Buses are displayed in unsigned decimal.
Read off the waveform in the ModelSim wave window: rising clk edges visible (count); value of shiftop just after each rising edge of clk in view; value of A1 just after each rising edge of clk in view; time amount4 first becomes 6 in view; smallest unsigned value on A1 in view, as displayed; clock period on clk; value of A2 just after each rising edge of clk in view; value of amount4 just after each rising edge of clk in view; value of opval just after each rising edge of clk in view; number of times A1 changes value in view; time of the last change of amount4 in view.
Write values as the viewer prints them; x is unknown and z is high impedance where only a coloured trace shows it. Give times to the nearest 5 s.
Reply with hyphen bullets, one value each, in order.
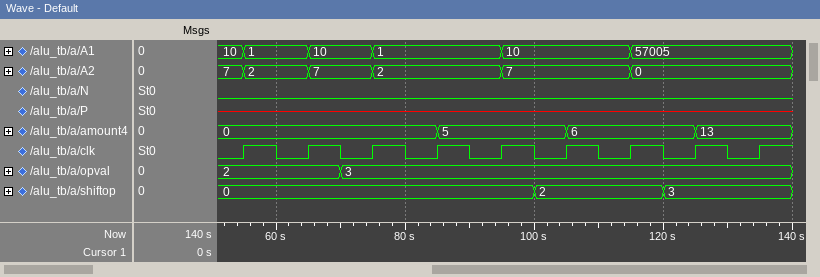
- 9
- 0, 0, 0, 0, 0, 2, 2, 3, 3
- 1, 10, 1, 1, 10, 10, 57005, 57005, 57005
- 105 s
- 1
- 10 s
- 2, 7, 2, 2, 7, 7, 0, 0, 0
- 0, 0, 0, 5, 5, 6, 6, 13, 13
- 2, 2, 3, 3, 3, 3, 3, 3, 3
- 5
- 125 s
